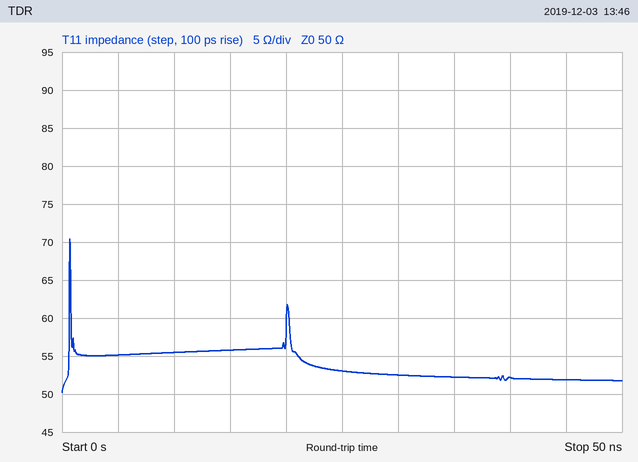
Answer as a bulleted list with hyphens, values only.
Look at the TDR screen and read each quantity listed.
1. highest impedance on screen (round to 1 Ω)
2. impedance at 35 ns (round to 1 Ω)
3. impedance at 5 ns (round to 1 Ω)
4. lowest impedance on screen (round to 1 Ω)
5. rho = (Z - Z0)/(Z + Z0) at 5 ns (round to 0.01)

- 70 Ω
- 52 Ω
- 55 Ω
- 50 Ω
- +0.05
